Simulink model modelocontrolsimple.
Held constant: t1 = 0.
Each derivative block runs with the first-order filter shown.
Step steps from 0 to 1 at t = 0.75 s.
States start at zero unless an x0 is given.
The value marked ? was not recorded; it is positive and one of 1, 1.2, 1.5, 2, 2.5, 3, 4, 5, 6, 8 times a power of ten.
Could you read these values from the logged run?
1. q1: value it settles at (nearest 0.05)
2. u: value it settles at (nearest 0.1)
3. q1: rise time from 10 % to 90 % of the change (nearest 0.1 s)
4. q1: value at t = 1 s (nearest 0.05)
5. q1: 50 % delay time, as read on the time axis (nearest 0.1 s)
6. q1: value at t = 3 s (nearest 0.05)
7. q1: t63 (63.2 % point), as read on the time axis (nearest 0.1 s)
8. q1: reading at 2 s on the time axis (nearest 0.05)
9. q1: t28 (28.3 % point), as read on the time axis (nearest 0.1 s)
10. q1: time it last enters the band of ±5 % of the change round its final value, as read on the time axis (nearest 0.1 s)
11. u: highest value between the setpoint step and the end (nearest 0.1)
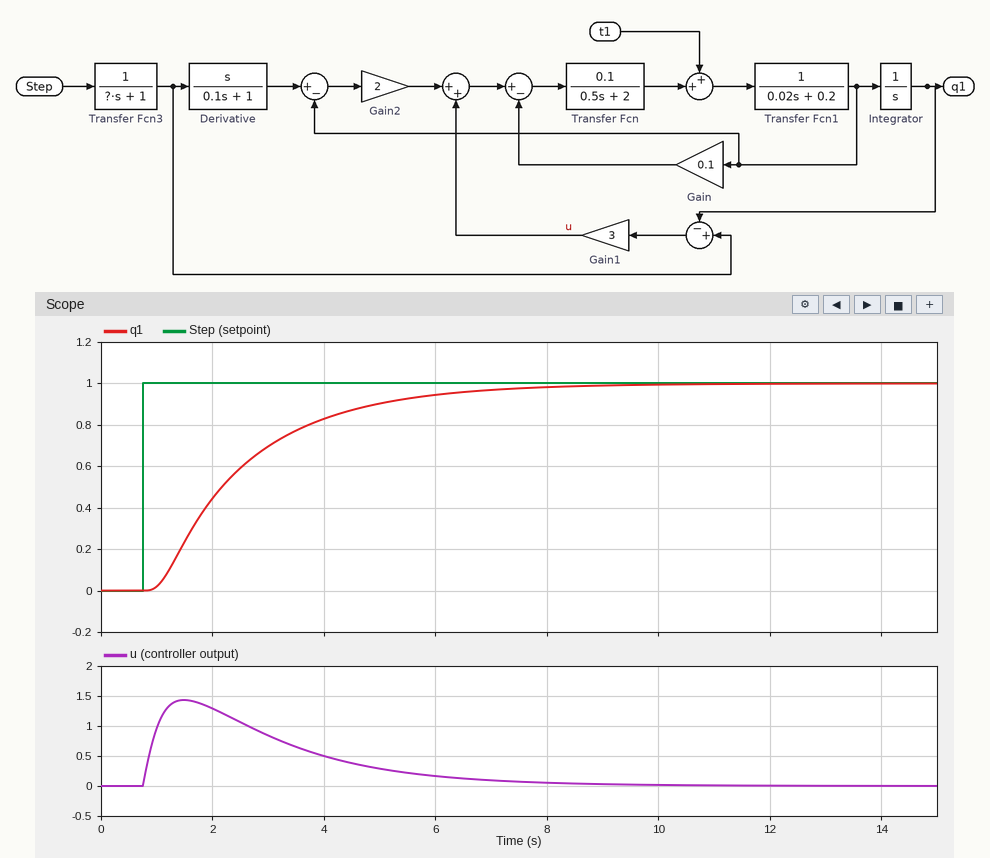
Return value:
1.00
0.0
3.7 s
0.00
2.2 s
0.70
2.7 s
0.45
1.6 s
6.2 s
1.4
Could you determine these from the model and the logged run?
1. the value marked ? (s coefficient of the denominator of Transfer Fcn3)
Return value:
0.6
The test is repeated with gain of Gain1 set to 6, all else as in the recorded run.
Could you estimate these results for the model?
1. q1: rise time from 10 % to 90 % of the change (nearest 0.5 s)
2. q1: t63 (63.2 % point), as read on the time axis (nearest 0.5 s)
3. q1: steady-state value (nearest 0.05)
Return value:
2.0 s
2.0 s
1.00
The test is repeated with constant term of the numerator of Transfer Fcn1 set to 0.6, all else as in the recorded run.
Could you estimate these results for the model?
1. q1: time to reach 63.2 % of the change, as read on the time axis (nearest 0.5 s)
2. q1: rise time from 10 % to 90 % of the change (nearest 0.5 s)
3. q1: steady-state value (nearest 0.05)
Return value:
3.5 s
5.5 s
1.00
